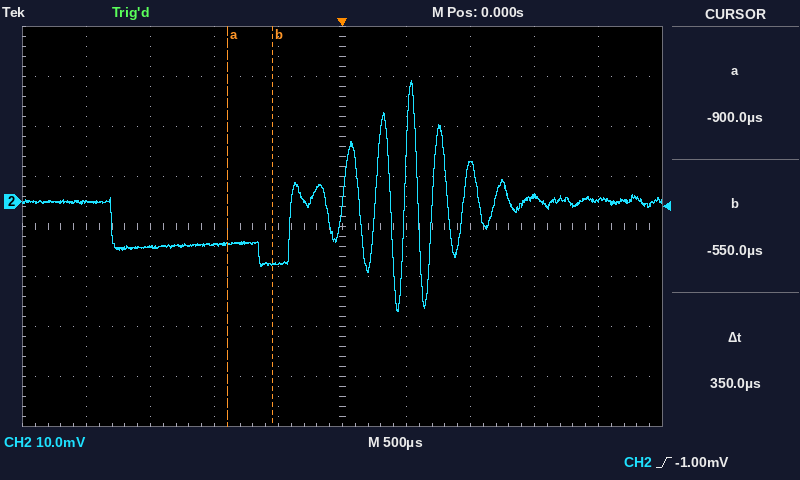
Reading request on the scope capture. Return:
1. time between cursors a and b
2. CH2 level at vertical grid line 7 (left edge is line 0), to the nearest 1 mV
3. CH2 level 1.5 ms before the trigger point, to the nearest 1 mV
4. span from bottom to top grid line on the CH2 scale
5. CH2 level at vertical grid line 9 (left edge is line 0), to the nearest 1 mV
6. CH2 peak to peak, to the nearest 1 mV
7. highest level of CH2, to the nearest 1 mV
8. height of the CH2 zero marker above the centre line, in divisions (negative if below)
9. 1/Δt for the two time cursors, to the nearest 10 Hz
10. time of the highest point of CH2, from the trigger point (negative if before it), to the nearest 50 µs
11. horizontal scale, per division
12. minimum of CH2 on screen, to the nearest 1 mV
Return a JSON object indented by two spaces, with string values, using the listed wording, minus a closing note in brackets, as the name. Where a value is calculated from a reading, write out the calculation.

{
  "time between cursors a and b": "350 µs",
  "CH2 level at vertical grid line 7 (left edge is line 0), to the nearest 1 mV": "7 mV",
  "CH2 level 1.5 ms before the trigger point, to the nearest 1 mV": "-9 mV",
  "span from bottom to top grid line on the CH2 scale": "80 mV",
  "CH2 level at vertical grid line 9 (left edge is line 0), to the nearest 1 mV": "0 mV",
  "CH2 peak to peak, to the nearest 1 mV": "24 mV − (-22 mV) = 46 mV",
  "highest level of CH2, to the nearest 1 mV": "24 mV",
  "height of the CH2 zero marker above the centre line, in divisions": "+0.5 div",
  "1/Δt for the two time cursors, to the nearest 10 Hz": "1 / 350 µs ≈ 2.86 kHz",
  "time of the highest point of CH2, from the trigger point (negative if before it), to the nearest 50 µs": "+550 µs",
  "horizontal scale, per division": "500 µs",
  "minimum of CH2 on screen, to the nearest 1 mV": "-22 mV"
}
